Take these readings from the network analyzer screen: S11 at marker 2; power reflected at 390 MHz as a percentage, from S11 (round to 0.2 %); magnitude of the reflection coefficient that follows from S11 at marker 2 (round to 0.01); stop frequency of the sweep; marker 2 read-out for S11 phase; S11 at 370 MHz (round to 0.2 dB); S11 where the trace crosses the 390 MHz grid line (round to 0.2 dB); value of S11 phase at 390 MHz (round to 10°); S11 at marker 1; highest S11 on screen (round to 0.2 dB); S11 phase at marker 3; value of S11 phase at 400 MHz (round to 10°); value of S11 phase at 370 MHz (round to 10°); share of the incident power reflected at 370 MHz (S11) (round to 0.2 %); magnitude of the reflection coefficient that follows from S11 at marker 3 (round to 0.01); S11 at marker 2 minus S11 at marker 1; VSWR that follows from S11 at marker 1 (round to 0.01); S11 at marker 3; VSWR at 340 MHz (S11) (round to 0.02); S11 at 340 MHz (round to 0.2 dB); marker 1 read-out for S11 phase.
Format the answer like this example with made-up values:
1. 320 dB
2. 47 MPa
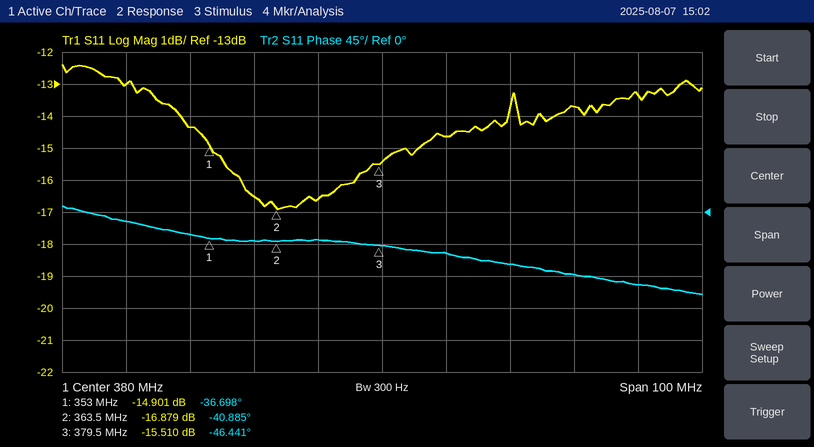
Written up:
1. -16.879 dB
2. 3.4 %
3. 0.14
4. 430 MHz
5. -40.885°
6. -16.6 dB
7. -14.6 dB
8. -60°
9. -14.901 dB
10. -12.4 dB
11. -46.441°
12. -70°
13. -40°
14. 2.2 %
15. 0.17
16. -1.978 dB
17. 1.44
18. -15.510 dB
19. 1.58
20. -13.0 dB
21. -36.698°
